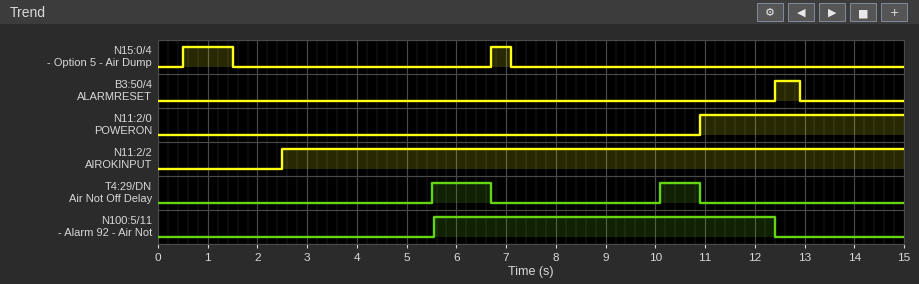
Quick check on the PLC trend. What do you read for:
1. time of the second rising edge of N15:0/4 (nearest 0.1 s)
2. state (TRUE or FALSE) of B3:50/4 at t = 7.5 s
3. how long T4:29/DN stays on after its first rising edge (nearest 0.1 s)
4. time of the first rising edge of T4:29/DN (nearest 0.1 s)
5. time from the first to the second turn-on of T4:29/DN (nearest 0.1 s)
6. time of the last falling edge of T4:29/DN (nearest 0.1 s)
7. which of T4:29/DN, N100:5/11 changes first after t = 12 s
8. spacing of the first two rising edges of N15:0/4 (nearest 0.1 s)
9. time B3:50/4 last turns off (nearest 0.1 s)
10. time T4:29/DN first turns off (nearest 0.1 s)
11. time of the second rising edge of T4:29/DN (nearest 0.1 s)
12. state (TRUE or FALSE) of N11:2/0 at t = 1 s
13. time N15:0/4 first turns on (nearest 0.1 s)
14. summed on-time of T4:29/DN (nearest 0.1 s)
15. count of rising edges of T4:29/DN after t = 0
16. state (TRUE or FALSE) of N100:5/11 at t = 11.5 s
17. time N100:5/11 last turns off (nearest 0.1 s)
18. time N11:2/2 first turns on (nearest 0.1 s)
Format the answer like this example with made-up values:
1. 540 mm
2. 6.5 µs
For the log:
1. 6.7 s
2. FALSE
3. 1.2 s
4. 5.5 s
5. 4.6 s
6. 10.9 s
7. N100:5/11
8. 6.2 s
9. 12.9 s
10. 6.7 s
11. 10.1 s
12. FALSE
13. 0.5 s
14. 2.0 s
15. 2
16. TRUE
17. 12.4 s
18. 2.5 s
